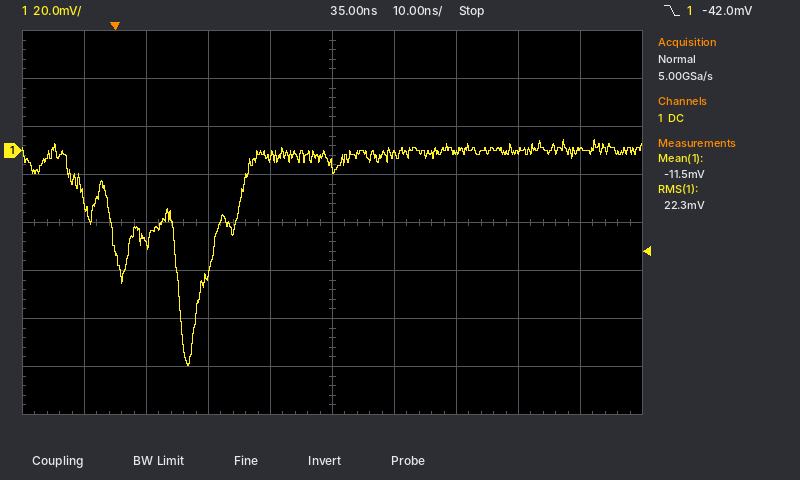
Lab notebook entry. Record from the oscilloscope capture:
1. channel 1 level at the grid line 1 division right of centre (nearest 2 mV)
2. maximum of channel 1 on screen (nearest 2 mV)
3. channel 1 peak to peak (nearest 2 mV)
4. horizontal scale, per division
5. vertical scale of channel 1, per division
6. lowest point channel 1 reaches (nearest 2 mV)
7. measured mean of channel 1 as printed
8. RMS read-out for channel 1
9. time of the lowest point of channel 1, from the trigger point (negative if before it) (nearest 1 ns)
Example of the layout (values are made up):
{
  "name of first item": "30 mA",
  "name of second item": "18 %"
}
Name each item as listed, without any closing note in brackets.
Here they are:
{
  "channel 1 level at the grid line 1 division right of centre": "-2 mV",
  "maximum of channel 1 on screen": "4 mV",
  "channel 1 peak to peak": "94 mV",
  "horizontal scale, per division": "10 ns",
  "vertical scale of channel 1, per division": "20 mV",
  "lowest point channel 1 reaches": "-90 mV",
  "measured mean of channel 1 as printed": "-11.5 mV",
  "RMS read-out for channel 1": "22.3 mV",
  "time of the lowest point of channel 1, from the trigger point (negative if before it)": "+12 ns"
}
